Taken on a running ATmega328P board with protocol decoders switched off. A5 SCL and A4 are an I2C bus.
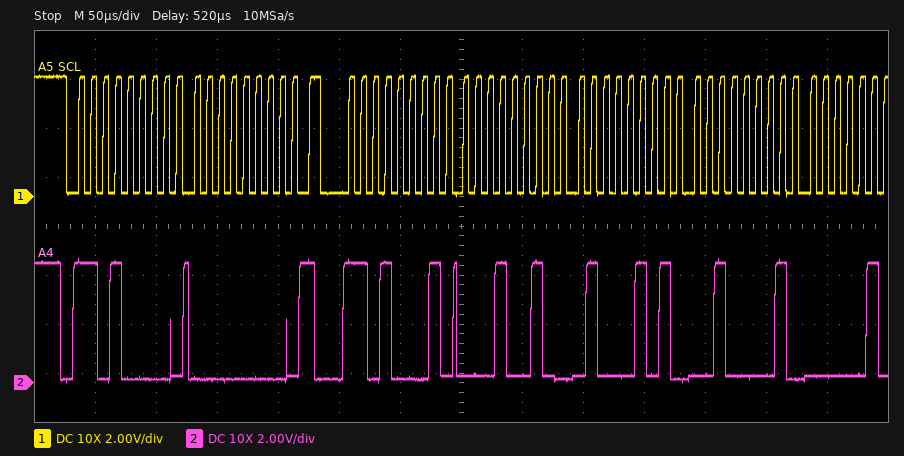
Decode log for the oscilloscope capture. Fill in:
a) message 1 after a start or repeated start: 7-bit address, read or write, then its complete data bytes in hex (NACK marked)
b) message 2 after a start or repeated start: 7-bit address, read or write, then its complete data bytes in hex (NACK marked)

0x68 write: 00
0x68 read: 12 45 21
